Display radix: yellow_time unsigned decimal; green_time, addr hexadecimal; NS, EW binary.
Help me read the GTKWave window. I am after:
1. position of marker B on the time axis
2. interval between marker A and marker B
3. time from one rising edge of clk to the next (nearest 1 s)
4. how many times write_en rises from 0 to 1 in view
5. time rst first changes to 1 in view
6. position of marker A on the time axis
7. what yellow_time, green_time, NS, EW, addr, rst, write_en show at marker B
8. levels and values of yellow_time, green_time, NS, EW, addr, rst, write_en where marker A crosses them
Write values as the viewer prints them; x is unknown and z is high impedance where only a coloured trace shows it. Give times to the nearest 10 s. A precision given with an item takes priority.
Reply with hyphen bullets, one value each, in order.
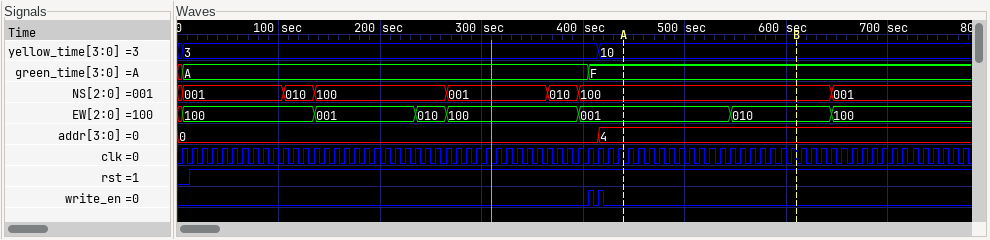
- 610 s
- 170 s
- 10 s
- 2
- 10 s
- 440 s
- yellow_time=10, green_time=F, NS=100, EW=010, addr=4, rst=1, write_en=0
- yellow_time=10, green_time=F, NS=100, EW=001, addr=4, rst=1, write_en=0
